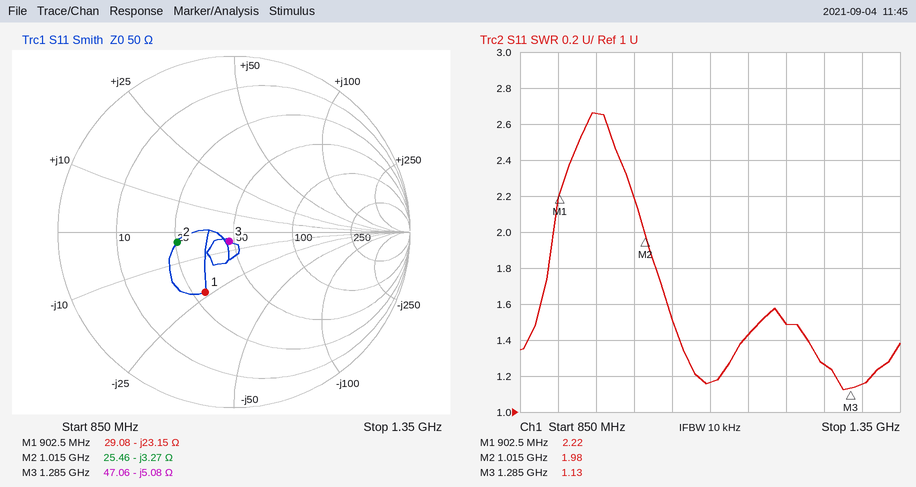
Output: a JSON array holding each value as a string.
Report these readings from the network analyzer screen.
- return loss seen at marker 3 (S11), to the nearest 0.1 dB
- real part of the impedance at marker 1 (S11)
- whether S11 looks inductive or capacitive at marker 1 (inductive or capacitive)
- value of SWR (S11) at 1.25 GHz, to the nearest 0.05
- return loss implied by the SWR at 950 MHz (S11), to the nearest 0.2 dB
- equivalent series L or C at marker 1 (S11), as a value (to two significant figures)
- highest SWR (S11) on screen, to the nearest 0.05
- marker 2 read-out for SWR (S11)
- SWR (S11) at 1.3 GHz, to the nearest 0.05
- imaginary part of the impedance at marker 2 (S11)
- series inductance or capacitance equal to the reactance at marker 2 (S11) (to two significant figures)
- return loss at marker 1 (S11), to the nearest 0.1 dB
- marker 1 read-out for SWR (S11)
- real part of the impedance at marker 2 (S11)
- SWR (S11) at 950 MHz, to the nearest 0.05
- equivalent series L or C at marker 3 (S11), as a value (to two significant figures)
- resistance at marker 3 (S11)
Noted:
["24.4 dB", "29.08 Ω", "capacitive", "1.25", "6.8 dB", "7.6 pF", "2.65", "1.98", "1.15", "-3.27 Ω", "48 pF", "8.4 dB", "2.22", "25.46 Ω", "2.65", "24 pF", "47.06 Ω"]
